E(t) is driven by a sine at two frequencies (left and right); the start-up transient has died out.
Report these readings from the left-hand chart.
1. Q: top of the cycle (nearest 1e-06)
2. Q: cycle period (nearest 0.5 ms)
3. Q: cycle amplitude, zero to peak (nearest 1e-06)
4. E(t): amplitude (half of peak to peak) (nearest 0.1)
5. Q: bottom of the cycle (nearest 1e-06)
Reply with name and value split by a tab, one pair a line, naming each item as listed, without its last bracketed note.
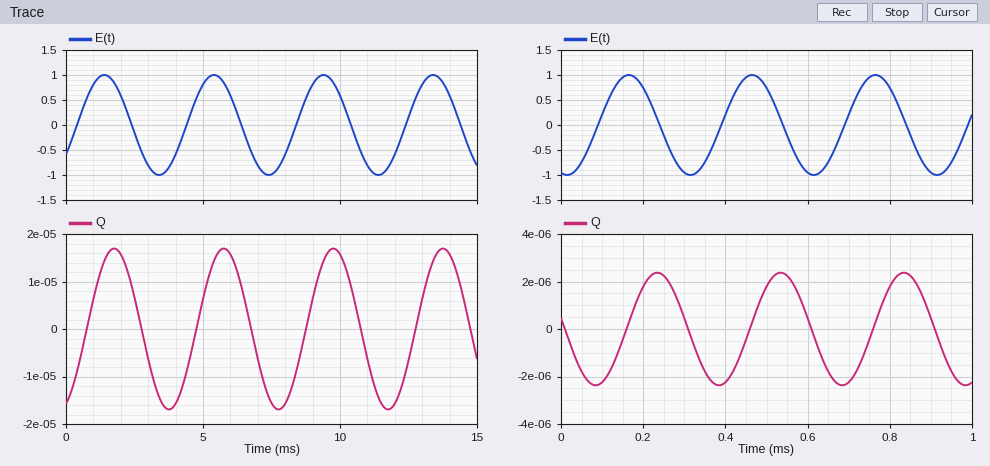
Q: top of the cycle	0.000017
Q: cycle period	4.0 ms
Q: cycle amplitude, zero to peak	0.000017
E(t): amplitude (half of peak to peak)	1.0
Q: bottom of the cycle	-0.000017
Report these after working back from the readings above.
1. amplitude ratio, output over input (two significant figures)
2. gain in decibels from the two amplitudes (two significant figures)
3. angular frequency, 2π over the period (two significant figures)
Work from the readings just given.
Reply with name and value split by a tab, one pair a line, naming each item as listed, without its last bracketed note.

amplitude ratio, output over input	0.000017
gain in decibels from the two amplitudes	-95 dB
angular frequency, 2π over the period	1.6 rad/ms
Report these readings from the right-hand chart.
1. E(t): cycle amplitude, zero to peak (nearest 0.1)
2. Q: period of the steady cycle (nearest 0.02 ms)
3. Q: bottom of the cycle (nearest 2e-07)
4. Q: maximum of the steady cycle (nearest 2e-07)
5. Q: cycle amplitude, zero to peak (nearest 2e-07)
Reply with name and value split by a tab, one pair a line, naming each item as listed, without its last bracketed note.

E(t): cycle amplitude, zero to peak	1.0
Q: period of the steady cycle	0.30 ms
Q: bottom of the cycle	-0.0000024
Q: maximum of the steady cycle	0.0000024
Q: cycle amplitude, zero to peak	0.0000024
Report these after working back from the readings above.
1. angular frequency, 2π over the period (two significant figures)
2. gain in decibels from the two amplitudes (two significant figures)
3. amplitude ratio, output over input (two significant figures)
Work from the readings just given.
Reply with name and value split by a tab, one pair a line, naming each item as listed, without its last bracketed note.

angular frequency, 2π over the period	21 rad/ms
gain in decibels from the two amplitudes	-110 dB
amplitude ratio, output over input	0.0000024
